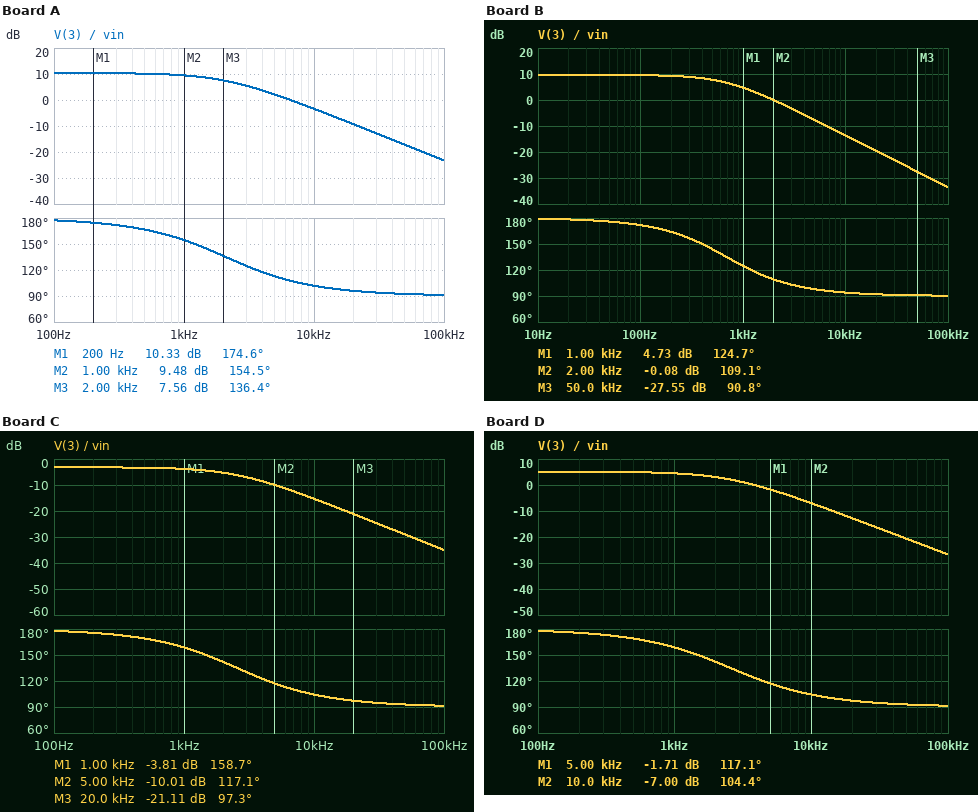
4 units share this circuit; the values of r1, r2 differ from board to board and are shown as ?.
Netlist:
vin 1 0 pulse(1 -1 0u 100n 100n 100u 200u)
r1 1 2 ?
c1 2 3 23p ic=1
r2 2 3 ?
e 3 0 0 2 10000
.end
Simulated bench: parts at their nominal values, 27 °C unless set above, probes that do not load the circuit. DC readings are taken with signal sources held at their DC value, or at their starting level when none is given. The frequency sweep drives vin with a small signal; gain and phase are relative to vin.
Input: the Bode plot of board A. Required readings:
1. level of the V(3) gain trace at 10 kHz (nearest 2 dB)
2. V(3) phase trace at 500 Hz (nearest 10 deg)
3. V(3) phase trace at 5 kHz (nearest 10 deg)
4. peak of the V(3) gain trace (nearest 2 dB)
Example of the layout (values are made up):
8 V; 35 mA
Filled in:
-4 dB; 170 deg; 110 deg; 10 dB
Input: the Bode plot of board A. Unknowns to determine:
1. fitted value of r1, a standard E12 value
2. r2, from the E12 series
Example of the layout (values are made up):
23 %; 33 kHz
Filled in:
1 MΩ; 3.3 MΩ
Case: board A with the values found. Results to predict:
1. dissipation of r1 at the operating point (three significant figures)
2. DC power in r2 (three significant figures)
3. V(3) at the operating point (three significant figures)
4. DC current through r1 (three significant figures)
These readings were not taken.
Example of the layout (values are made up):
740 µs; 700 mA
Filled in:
999 nW; 3.30 µW; -3.30 V; 1.00 µA
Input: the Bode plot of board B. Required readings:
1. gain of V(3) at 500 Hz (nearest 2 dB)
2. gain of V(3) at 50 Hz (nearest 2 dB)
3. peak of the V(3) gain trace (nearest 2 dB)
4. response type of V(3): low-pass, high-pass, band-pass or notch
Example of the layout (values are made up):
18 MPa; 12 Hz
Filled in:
8 dB; 10 dB; 10 dB; low-pass
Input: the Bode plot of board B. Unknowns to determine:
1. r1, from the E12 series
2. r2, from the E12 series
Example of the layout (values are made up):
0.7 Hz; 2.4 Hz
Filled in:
3.3 MΩ; 10 MΩ
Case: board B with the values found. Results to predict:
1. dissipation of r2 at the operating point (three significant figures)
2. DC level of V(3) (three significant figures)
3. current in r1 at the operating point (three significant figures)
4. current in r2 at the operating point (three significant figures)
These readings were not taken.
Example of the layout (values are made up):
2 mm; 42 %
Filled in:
918 nW; -3.03 V; 303 nA; 303 nA
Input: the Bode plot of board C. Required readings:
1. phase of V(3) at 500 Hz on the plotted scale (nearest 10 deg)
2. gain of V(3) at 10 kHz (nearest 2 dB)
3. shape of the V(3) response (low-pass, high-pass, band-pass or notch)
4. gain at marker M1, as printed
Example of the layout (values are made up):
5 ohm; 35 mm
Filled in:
170 deg; -16 dB; low-pass; -3.81 dB
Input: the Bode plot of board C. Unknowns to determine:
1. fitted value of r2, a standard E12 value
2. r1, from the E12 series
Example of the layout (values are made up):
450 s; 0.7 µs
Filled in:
2.7 MΩ; 3.9 MΩ
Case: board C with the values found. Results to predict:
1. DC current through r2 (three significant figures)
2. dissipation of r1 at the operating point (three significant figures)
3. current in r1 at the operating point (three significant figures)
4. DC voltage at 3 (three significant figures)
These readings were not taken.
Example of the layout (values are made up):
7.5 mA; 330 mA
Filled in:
256 nA; 256 nW; 256 nA; -692 mV
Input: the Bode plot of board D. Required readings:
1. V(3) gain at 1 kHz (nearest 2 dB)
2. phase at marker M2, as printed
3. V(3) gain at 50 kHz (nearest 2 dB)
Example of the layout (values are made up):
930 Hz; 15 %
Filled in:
4 dB; 104.4 deg; -20 dB
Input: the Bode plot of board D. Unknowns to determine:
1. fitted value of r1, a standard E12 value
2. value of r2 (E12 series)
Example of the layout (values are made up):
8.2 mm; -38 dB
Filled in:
1.5 MΩ; 2.7 MΩ
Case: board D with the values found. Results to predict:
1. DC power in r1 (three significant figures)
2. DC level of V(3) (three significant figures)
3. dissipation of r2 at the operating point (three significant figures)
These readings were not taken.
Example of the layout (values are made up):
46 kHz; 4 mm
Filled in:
666 nW; -1.80 V; 1.20 µW
